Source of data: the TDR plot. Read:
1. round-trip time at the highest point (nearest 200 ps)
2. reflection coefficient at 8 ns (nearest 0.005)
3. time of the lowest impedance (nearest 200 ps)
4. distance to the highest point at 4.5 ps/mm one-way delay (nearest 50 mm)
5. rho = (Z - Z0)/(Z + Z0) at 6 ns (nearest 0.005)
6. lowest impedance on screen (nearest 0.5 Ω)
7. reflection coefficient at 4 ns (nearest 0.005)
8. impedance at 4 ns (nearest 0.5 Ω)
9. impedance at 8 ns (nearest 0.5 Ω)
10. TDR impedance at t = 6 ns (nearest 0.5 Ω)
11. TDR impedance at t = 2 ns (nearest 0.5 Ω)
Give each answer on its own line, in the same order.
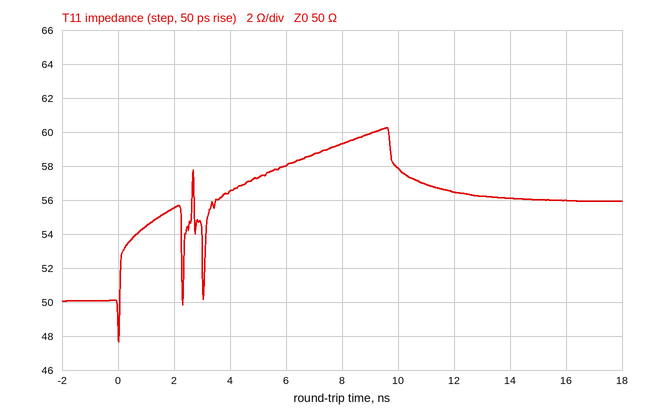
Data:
9.6 ns
+0.085
0.0 ns
1.05 m
+0.075
47.5 Ω
+0.060
56.5 Ω
59.5 Ω
58.0 Ω
55.5 Ω
